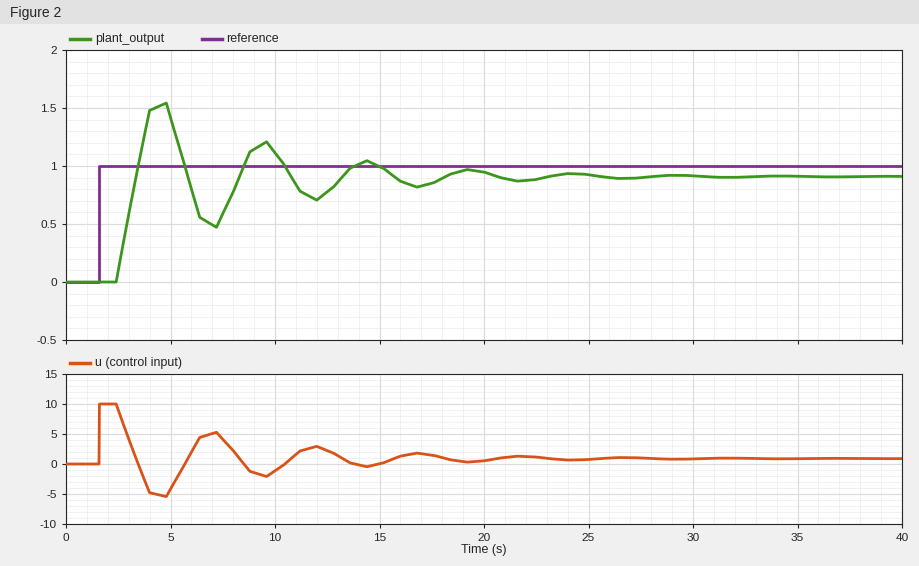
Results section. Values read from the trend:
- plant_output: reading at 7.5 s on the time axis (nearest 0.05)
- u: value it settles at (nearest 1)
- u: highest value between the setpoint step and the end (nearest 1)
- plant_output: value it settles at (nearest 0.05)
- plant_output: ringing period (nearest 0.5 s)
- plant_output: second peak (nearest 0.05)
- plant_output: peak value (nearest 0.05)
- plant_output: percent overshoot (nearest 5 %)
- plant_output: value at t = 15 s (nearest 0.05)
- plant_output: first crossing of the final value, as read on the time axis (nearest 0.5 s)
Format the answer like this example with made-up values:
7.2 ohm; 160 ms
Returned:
0.60; 1; 10; 0.90; 5.0 s; 1.20; 1.55; 70 %; 1.00; 3.5 s
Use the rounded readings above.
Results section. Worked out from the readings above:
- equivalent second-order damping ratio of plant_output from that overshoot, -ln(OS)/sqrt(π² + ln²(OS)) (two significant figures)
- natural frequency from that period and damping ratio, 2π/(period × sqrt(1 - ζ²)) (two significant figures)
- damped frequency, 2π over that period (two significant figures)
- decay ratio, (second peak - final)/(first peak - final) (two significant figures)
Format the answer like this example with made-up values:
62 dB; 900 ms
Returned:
0.11; 1.3 rad/s; 1.3 rad/s; 0.46
